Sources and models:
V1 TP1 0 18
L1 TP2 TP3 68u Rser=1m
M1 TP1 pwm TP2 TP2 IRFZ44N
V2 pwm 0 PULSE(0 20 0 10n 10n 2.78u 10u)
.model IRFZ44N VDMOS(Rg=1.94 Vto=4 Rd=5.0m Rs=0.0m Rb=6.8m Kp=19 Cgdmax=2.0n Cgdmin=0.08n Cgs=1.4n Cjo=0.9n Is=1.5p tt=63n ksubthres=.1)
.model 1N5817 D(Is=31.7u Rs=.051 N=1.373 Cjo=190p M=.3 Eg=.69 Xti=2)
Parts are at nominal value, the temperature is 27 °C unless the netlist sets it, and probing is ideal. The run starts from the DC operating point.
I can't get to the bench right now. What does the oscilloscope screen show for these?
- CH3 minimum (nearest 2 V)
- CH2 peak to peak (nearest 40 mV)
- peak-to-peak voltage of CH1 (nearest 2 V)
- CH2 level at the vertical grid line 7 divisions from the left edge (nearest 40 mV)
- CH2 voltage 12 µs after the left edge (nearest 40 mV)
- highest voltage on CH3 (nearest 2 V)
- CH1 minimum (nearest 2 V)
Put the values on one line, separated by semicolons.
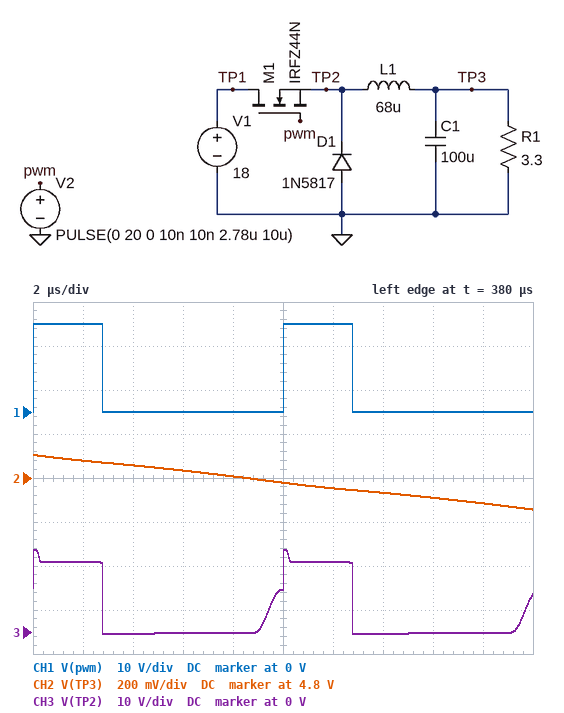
0 V; 240 mV; 20 V; 4.72 V; 4.76 V; 18 V; 0 V
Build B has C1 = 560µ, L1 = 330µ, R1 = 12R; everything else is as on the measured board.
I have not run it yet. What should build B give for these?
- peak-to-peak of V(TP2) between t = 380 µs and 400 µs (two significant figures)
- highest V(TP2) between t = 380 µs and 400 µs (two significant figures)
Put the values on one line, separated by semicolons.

16 V; 15 V
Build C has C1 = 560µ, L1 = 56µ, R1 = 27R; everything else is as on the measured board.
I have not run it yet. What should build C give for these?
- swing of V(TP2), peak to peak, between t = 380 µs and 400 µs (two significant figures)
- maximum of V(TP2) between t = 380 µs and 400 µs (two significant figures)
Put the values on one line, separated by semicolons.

16 V; 15 V
